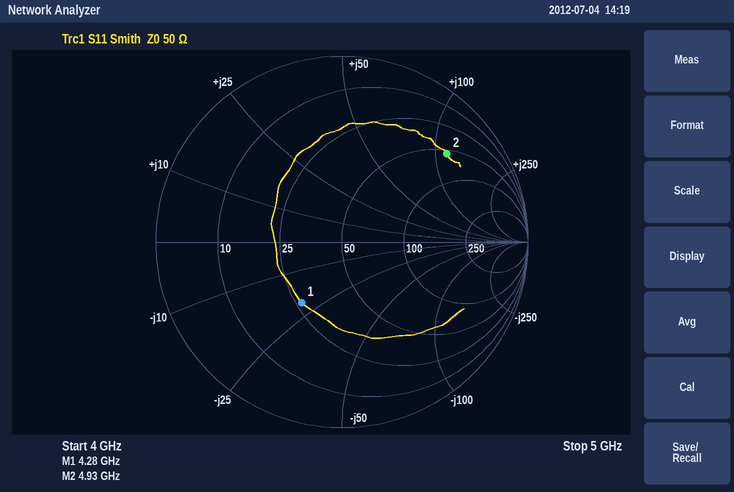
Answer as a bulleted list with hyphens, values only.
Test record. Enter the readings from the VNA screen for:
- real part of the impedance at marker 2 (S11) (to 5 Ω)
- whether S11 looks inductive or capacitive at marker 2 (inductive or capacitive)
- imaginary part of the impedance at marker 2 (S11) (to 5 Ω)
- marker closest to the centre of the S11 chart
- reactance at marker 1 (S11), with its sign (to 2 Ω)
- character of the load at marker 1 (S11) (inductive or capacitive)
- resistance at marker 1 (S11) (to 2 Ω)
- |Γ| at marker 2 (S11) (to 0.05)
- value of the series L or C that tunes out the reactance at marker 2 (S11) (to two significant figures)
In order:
- 55 Ω
- inductive
- +115 Ω
- marker 1
- -20 Ω
- capacitive
- 26 Ω
- 0.75
- 280 fF
